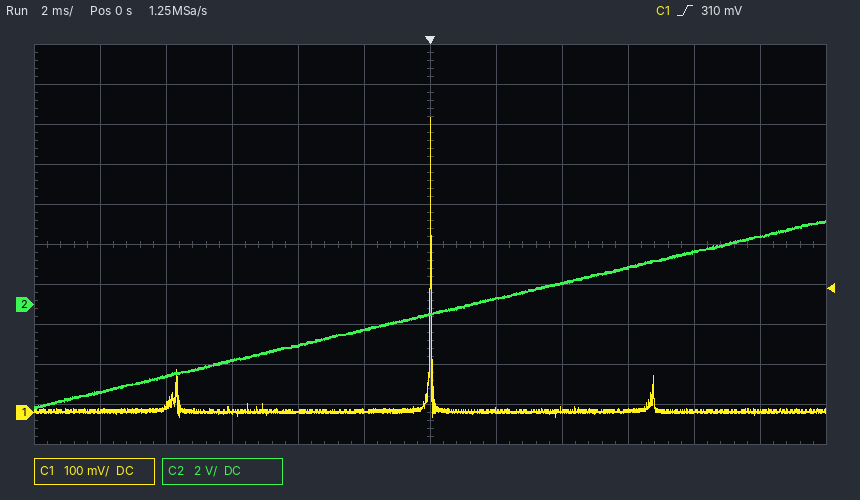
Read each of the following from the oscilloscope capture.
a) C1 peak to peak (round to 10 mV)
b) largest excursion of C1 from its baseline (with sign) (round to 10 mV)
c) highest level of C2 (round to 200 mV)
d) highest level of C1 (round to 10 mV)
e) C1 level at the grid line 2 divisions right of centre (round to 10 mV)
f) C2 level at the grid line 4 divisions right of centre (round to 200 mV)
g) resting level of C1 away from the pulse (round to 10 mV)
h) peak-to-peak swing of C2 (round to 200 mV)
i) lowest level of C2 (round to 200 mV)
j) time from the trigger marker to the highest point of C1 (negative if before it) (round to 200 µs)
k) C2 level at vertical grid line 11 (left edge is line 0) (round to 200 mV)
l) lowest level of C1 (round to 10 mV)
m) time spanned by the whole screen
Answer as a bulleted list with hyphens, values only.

- 750 mV
- +740 mV
- 4.2 V
- 740 mV
- 10 mV
- 2.6 V
- 0 mV
- 9.4 V
- -5.2 V
- 0.0 ms
- 3.4 V
- -10 mV
- 24 ms
